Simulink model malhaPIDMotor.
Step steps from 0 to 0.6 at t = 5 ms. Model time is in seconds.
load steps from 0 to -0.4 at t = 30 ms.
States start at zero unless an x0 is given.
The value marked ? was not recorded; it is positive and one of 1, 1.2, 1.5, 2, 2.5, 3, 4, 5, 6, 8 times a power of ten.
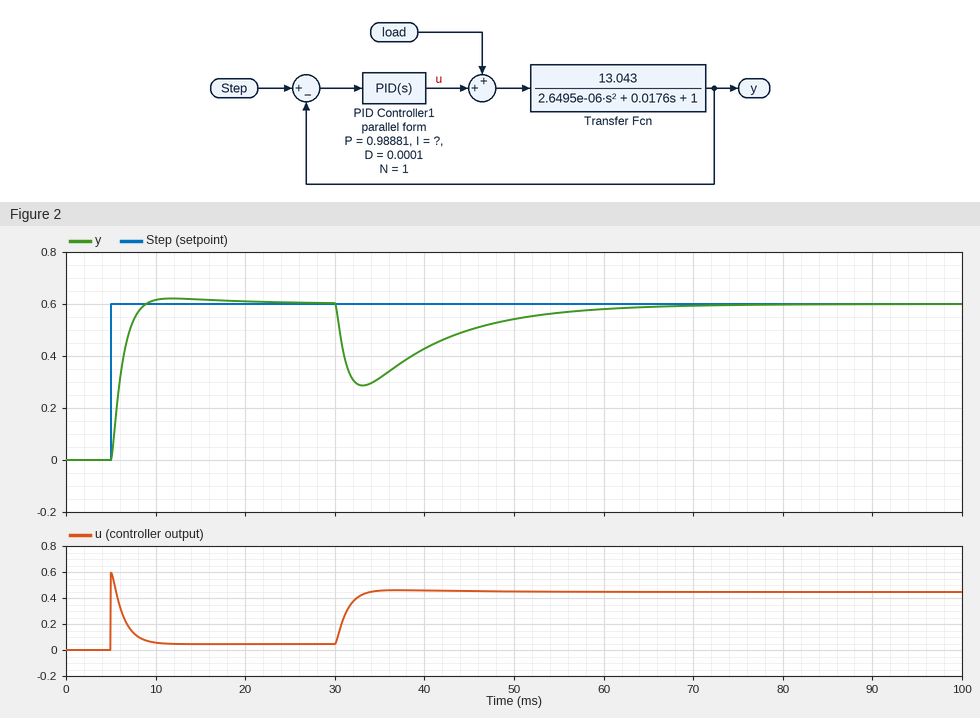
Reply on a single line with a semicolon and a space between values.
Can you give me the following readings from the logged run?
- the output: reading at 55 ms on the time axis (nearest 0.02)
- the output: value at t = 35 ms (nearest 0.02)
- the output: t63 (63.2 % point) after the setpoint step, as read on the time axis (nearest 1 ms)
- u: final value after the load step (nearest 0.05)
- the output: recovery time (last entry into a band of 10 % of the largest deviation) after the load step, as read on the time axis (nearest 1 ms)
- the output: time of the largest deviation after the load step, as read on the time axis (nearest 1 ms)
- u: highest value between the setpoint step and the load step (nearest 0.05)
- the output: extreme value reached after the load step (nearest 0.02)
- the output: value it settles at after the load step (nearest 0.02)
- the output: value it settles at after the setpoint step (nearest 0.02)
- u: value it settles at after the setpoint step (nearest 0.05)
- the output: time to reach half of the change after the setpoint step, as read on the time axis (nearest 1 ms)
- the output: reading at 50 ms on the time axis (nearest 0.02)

0.56; 0.32; 6 ms; 0.45; 56 ms; 33 ms; 0.60; 0.28; 0.60; 0.60; 0.05; 6 ms; 0.54
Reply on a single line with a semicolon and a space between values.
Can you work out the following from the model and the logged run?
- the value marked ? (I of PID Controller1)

100
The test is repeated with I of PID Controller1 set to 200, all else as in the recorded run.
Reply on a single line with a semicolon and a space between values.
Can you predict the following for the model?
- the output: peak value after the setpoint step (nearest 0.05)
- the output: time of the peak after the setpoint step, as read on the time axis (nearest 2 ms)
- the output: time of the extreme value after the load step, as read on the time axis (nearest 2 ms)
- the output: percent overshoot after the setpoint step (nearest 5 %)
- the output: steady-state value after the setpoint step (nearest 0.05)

0.65; 10 ms; 32 ms; 10 %; 0.60
